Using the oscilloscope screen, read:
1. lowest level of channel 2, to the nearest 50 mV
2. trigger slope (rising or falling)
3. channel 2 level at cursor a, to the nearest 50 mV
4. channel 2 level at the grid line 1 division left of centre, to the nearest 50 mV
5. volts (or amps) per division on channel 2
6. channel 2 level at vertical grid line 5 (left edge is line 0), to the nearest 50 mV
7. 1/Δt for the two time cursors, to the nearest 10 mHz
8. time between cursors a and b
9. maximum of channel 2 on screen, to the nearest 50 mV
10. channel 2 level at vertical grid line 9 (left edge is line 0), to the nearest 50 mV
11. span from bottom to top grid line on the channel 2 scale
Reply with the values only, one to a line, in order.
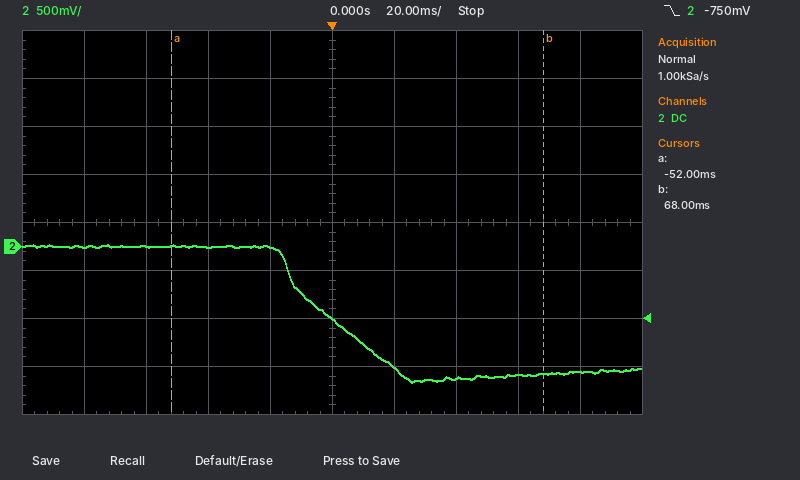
-1.40 V
falling
0 mV
0 mV
500 mV
-750 mV
8.33 Hz
120 ms
0 mV
-1.30 V
4 V
